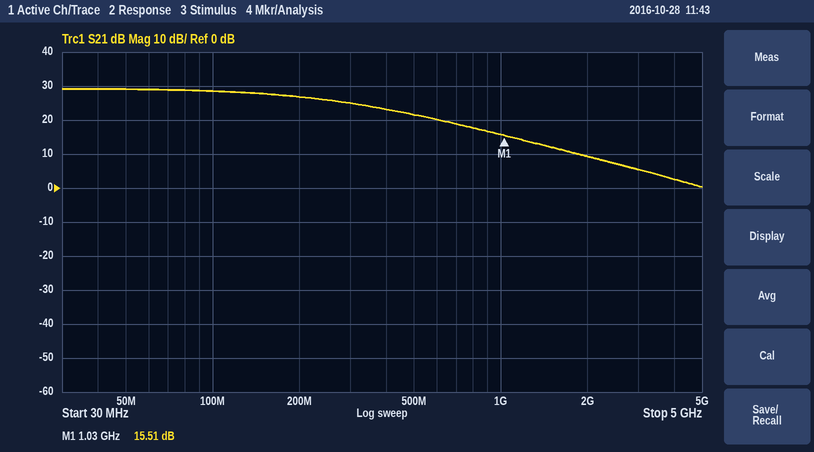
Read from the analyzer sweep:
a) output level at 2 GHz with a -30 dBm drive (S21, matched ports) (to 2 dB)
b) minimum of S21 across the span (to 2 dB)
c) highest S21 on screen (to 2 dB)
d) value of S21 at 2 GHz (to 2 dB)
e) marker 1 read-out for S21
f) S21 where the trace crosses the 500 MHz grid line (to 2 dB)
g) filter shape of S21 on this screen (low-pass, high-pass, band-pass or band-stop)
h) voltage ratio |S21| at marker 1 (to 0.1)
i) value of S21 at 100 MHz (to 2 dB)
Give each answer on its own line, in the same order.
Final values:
-20 dBm
0 dB
30 dB
10 dB
15.51 dB
22 dB
low-pass
6.0
28 dB
